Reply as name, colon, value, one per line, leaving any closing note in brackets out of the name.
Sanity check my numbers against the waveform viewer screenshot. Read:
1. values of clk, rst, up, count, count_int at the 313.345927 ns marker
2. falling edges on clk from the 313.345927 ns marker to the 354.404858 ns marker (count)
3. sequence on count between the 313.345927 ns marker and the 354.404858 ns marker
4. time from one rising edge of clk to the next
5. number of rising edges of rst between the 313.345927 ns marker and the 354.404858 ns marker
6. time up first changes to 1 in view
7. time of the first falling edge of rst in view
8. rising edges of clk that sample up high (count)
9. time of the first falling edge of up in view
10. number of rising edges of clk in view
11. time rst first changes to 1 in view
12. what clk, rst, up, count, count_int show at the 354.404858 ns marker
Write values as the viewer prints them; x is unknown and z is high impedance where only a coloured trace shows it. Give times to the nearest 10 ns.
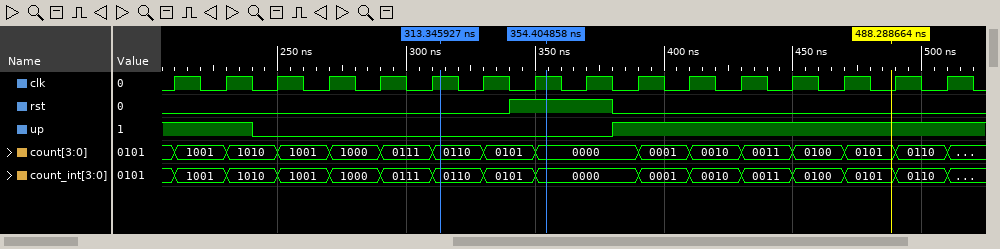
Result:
values of clk, rst, up, count, count_int at the 313.345927 ns marker: clk=1, rst=0, up=0, count=0110, count_int=0110
falling edges on clk from the 313.345927 ns marker to the 354.404858 ns marker: 2
sequence on count between the 313.345927 ns marker and the 354.404858 ns marker: 0110, 0101, 0000
time from one rising edge of clk to the next: 20 ns
number of rising edges of rst between the 313.345927 ns marker and the 354.404858 ns marker: 1
time up first changes to 1 in view: 380 ns
time of the first falling edge of rst in view: 380 ns
rising edges of clk that sample up high: 9
time of the first falling edge of up in view: 240 ns
number of rising edges of clk in view: 16
time rst first changes to 1 in view: 340 ns
what clk, rst, up, count, count_int show at the 354.404858 ns marker: clk=1, rst=1, up=0, count=0000, count_int=0000
